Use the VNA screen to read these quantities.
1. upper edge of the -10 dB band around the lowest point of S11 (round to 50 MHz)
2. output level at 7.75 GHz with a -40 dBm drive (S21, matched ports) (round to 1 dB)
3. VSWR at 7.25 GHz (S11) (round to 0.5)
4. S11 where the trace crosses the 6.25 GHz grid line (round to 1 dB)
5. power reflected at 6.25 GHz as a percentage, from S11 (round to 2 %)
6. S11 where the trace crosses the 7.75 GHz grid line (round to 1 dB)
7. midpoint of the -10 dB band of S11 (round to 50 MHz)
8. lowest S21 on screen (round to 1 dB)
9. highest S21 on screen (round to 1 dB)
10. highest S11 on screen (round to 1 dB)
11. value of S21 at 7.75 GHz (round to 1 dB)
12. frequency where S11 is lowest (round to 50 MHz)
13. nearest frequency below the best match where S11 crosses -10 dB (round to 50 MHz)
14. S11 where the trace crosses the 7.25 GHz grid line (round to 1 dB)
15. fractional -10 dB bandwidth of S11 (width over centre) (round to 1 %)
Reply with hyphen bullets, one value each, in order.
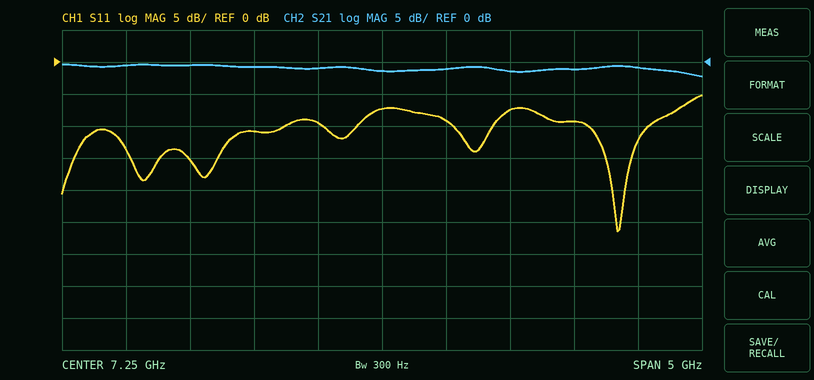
- 9.35 GHz
- -41 dBm
- 2.5
- -11 dB
- 8 %
- -9 dB
- 9.10 GHz
- -2 dB
- 0 dB
- -5 dB
- -1 dB
- 9.10 GHz
- 8.85 GHz
- -7 dB
- 5 %
